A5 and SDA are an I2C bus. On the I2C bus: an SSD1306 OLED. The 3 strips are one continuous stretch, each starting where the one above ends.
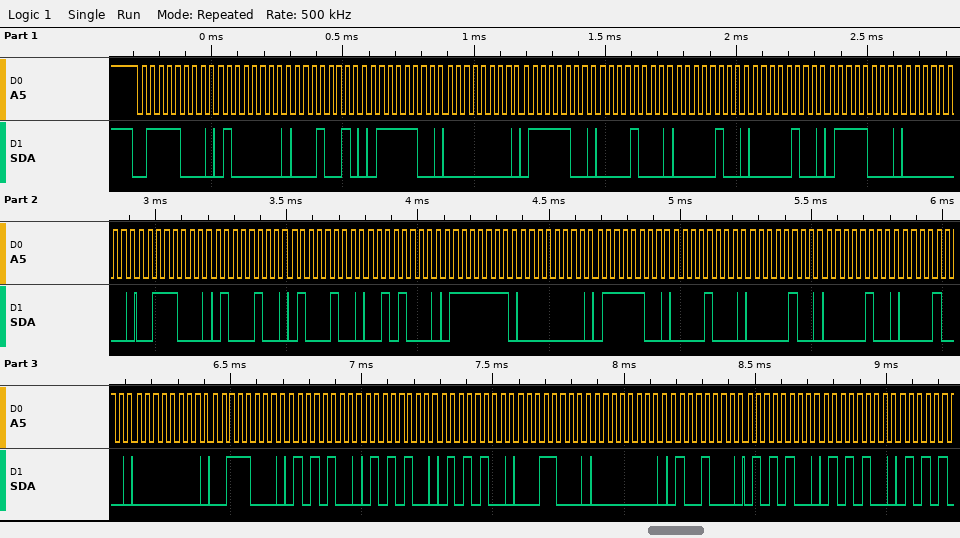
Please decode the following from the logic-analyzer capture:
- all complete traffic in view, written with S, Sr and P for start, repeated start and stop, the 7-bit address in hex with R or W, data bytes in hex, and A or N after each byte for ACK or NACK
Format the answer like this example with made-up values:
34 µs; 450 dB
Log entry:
S 3CW A 40 A 12 A 7C A 00 A 7C A 08 A 04 A 04 A 78 A 00 A 38 A 44 A 44 A 28 A 7F A 00 A 7C A 08 A 04 A 04 A 08 A 00 A 38 A 54 A 54 A 54 A 18 A 00 A 48 A 54 A 54 A
